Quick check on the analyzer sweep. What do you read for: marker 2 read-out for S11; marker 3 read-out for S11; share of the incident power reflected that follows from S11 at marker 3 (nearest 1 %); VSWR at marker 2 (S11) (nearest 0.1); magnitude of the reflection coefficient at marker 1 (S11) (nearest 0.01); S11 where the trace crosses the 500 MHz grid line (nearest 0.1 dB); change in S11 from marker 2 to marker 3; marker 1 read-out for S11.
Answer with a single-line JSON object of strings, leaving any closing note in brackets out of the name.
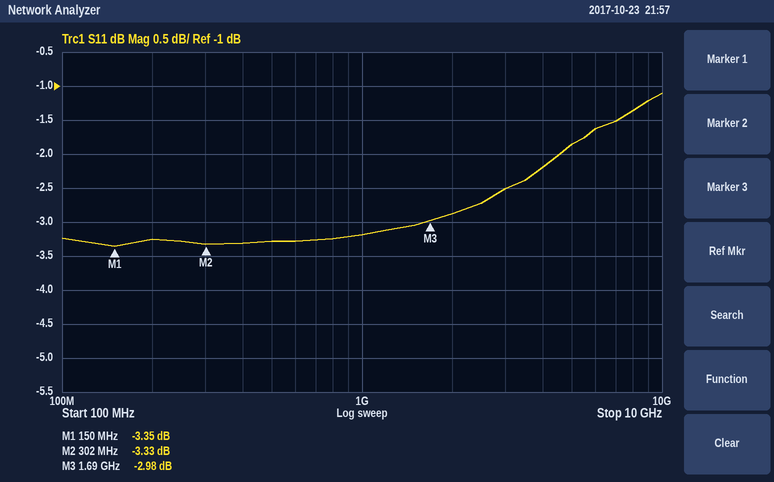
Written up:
{"marker 2 read-out for S11": "-3.33 dB", "marker 3 read-out for S11": "-2.98 dB", "share of the incident power reflected that follows from S11 at marker 3": "50 %", "VSWR at marker 2 (S11)": "5.3", "magnitude of the reflection coefficient at marker 1 (S11)": "0.68", "S11 where the trace crosses the 500 MHz grid line": "-3.3 dB", "change in S11 from marker 2 to marker 3": "0.35 dB", "marker 1 read-out for S11": "-3.35 dB"}
